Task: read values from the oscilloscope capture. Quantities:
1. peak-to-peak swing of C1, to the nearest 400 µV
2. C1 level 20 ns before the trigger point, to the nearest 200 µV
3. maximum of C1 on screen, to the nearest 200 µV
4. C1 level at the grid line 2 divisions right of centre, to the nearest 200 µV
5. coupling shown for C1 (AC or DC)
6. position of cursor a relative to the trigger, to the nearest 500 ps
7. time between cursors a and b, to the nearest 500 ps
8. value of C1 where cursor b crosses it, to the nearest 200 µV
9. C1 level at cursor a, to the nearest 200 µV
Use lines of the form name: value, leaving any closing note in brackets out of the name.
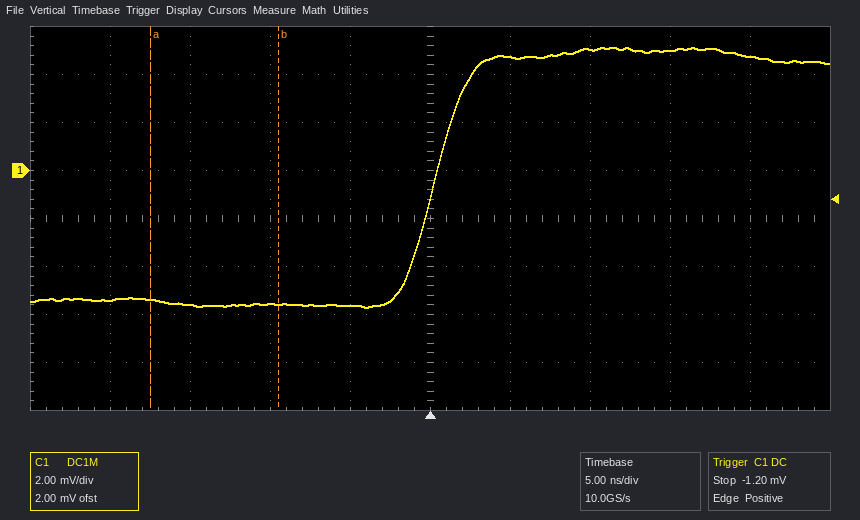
peak-to-peak swing of C1, to the nearest 400 µV: 10.8 mV
C1 level 20 ns before the trigger point, to the nearest 200 µV: -5.4 mV
maximum of C1 on screen, to the nearest 200 µV: 5.2 mV
C1 level at the grid line 2 divisions right of centre, to the nearest 200 µV: 5.0 mV
coupling shown for C1: DC
position of cursor a relative to the trigger, to the nearest 500 ps: -17.5 ns
time between cursors a and b, to the nearest 500 ps: 8.0 ns
value of C1 where cursor b crosses it, to the nearest 200 µV: -5.6 mV
C1 level at cursor a, to the nearest 200 µV: -5.4 mV
